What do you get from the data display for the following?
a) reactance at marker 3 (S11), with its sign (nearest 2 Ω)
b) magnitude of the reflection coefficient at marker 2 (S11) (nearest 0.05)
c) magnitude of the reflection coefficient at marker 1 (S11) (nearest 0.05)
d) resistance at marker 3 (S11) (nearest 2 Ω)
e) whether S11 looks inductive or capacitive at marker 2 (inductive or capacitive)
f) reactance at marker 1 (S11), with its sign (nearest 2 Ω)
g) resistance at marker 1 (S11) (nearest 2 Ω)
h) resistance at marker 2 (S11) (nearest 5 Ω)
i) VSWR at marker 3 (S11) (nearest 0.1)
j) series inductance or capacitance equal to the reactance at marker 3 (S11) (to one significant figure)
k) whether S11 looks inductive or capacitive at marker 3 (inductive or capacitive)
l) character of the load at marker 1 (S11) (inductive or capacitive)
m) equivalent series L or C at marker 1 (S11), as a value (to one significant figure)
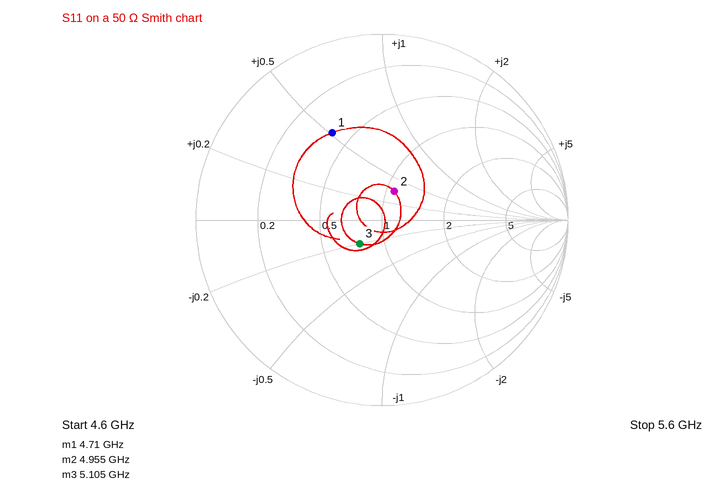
-10 Ω
0.15
0.55
38 Ω
inductive
+26 Ω
20 Ω
55 Ω
1.4
3 pF
capacitive
inductive
900 pH
